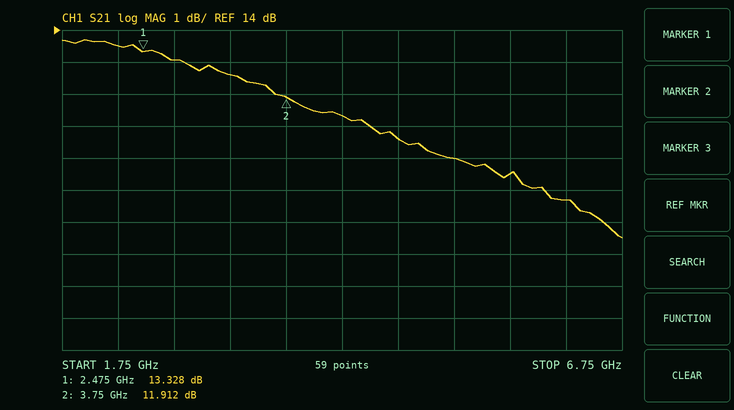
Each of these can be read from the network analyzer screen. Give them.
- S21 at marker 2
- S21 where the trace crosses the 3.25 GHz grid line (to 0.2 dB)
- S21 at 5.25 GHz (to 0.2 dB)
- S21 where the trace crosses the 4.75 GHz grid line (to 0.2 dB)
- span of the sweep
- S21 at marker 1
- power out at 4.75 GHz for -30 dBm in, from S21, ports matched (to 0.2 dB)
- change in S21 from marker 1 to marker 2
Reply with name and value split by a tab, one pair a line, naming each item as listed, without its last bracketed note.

S21 at marker 2	11.912 dB
S21 where the trace crosses the 3.25 GHz grid line	12.6 dB
S21 at 5.25 GHz	10.0 dB
S21 where the trace crosses the 4.75 GHz grid line	10.6 dB
span of the sweep	5 GHz
S21 at marker 1	13.328 dB
power out at 4.75 GHz for -30 dBm in, from S21, ports matched	-19.4 dBm
change in S21 from marker 1 to marker 2	-1.416 dB
